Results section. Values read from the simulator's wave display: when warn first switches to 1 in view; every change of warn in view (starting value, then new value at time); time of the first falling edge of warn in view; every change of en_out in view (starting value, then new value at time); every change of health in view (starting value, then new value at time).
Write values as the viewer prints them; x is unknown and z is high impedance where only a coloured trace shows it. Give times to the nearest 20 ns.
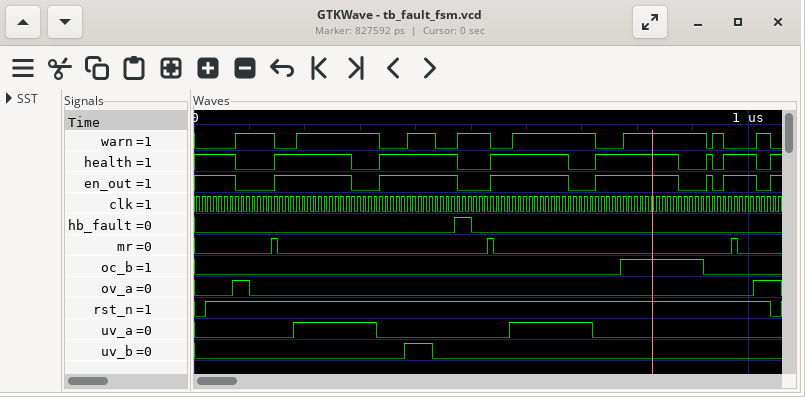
80 ns
0, 1 at 80 ns, 0 at 140 ns, 1 at 180 ns, 0 at 340 ns, 1 at 380 ns, 0 at 440 ns, 1 at 480 ns, 0 at 540 ns, 1 at 580 ns, 0 at 720 ns, 1 at 780 ns, 0 at 920 ns, 1 at 940 ns, 0 at 960 ns, 1 at 1020 ns, 0 at 1040 ns
140 ns
1, 0 at 80 ns, 1 at 140 ns, 0 at 280 ns, 1 at 340 ns, 0 at 480 ns, 1 at 540 ns, 0 at 680 ns, 1 at 720 ns, 0 at 880 ns, 1 at 920 ns, 0 at 940 ns, 1 at 960 ns, 0 at 1020 ns, 1 at 1040 ns
1, 0 at 80 ns, 1 at 140 ns, 0 at 280 ns, 1 at 340 ns, 0 at 480 ns, 1 at 540 ns, 0 at 680 ns, 1 at 720 ns, 0 at 880 ns, 1 at 920 ns, 0 at 940 ns, 1 at 960 ns, 0 at 1020 ns, 1 at 1040 ns
